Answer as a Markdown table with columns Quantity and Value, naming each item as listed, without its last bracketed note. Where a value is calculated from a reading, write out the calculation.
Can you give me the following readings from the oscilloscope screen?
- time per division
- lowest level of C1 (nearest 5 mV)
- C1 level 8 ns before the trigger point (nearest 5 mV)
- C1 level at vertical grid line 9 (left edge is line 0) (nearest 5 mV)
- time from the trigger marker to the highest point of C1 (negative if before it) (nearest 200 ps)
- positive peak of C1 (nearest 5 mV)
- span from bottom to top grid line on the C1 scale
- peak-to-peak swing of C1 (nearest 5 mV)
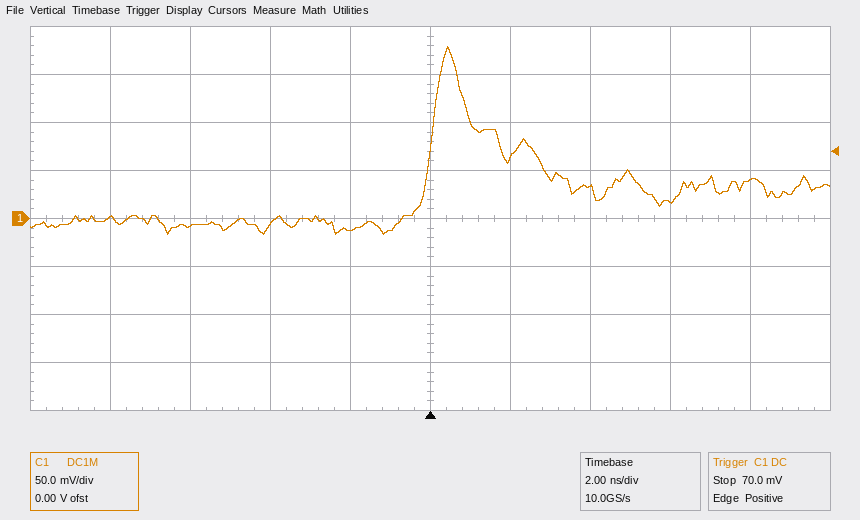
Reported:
| Quantity | Value |
|---|---|
| time per division | 2 ns |
| lowest level of C1 | -15 mV |
| C1 level 8 ns before the trigger point | 0 mV |
| C1 level at vertical grid line 9 (left edge is line 0) | 40 mV |
| time from the trigger marker to the highest point of C1 (negative if before it) | +400 ps |
| positive peak of C1 | 180 mV |
| span from bottom to top grid line on the C1 scale | 400 mV |
| peak-to-peak swing of C1 | 180 mV − (-15 mV) = 195 mV |
